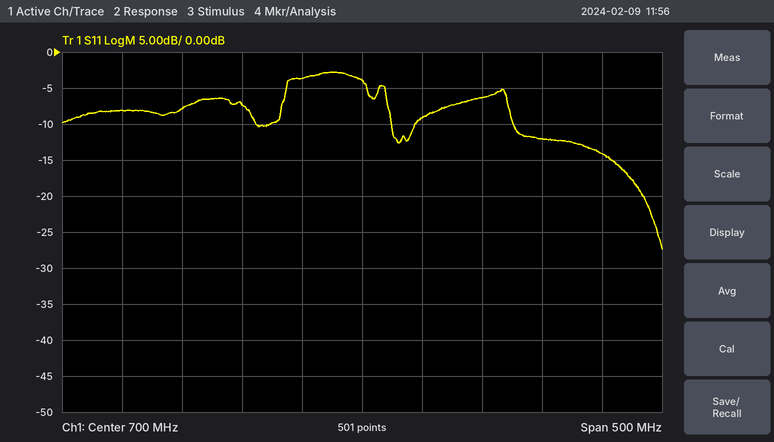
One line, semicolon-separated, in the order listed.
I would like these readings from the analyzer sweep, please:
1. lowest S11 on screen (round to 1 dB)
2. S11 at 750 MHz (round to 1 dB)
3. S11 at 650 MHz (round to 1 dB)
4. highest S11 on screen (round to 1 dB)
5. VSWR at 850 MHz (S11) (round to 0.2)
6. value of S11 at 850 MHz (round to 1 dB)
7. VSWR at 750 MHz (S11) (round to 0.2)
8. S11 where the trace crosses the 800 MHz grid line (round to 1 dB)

-27 dB; -9 dB; -4 dB; -3 dB; 1.6; -12 dB; 2.0; -6 dB
